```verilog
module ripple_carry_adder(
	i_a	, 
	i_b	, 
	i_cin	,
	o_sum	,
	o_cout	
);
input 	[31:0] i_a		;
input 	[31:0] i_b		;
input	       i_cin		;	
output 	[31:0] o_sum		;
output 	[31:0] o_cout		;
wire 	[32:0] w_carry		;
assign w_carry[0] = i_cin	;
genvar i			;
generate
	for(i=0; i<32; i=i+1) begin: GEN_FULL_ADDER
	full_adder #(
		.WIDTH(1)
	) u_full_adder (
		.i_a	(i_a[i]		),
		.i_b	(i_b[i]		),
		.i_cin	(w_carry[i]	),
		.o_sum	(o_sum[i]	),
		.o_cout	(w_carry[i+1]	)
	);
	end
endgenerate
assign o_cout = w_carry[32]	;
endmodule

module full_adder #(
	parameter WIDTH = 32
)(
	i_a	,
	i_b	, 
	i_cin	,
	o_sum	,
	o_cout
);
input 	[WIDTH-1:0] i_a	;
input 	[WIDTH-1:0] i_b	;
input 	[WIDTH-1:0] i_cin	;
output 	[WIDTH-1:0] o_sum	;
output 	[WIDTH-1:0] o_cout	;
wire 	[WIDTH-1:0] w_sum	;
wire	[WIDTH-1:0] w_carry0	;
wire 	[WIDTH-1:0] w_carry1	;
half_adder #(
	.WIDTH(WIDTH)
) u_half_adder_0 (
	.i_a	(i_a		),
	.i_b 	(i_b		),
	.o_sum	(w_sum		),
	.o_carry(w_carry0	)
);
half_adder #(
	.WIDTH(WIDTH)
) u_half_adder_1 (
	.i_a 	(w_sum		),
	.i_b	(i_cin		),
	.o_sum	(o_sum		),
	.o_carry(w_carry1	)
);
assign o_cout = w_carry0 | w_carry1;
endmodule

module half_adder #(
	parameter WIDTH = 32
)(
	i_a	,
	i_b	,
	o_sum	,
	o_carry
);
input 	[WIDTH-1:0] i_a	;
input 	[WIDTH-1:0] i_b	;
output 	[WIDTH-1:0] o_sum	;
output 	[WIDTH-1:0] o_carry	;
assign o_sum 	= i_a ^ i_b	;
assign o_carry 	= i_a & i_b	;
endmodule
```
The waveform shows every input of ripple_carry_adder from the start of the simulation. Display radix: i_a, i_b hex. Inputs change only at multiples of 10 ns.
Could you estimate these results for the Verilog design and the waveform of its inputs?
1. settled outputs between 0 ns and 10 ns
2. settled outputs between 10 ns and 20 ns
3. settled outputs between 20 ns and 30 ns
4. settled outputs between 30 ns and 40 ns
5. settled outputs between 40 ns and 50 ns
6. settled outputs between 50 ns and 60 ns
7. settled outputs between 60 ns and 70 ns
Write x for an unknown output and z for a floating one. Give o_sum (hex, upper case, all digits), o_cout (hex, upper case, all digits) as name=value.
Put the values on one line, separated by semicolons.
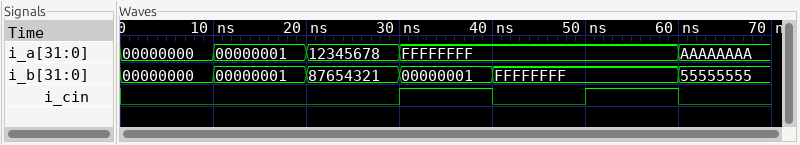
o_sum=00000000, o_cout=00000000; o_sum=00000002, o_cout=00000000; o_sum=99999999, o_cout=00000000; o_sum=00000001, o_cout=00000001; o_sum=FFFFFFFE, o_cout=00000001; o_sum=FFFFFFFF, o_cout=00000001; o_sum=FFFFFFFF, o_cout=00000000
